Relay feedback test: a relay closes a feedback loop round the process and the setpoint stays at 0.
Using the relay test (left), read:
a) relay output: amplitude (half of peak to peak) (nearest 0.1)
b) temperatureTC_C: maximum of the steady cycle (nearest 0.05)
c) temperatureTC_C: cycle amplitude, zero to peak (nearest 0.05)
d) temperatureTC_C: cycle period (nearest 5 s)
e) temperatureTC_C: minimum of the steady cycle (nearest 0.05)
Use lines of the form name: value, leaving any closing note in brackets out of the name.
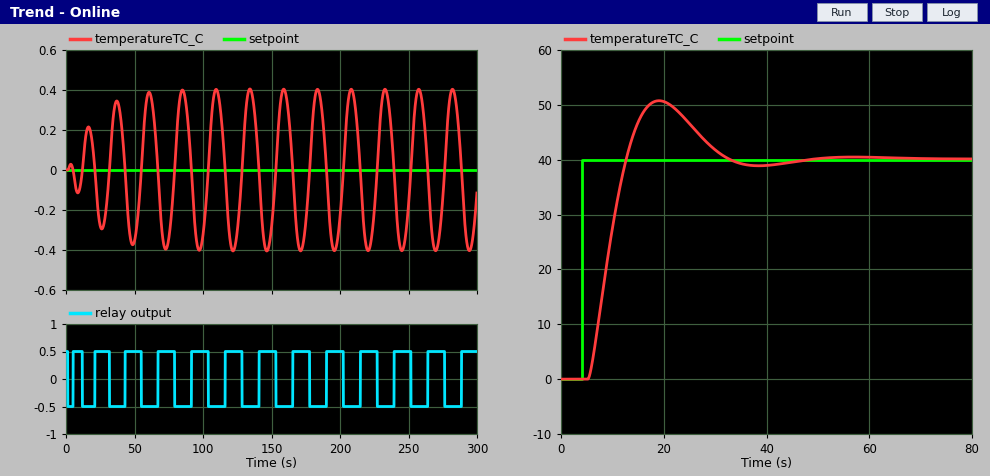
relay output: amplitude (half of peak to peak): 0.5
temperatureTC_C: maximum of the steady cycle: 0.40
temperatureTC_C: cycle amplitude, zero to peak: 0.40
temperatureTC_C: cycle period: 25 s
temperatureTC_C: minimum of the steady cycle: -0.40
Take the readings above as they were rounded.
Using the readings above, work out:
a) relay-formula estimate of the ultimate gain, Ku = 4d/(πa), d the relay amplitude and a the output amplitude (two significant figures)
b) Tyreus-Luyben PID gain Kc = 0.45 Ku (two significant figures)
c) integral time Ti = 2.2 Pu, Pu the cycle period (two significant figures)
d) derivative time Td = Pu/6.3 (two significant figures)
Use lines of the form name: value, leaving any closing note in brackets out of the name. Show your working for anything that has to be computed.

relay-formula estimate of the ultimate gain, Ku = 4d/(πa), d the relay amplitude and a the output amplitude: 4 × 0.5 / (π × 0.4) = 1.6
Tyreus-Luyben PID gain Kc = 0.45 Ku: 0.45 × 1.6 = 0.72
integral time Ti = 2.2 Pu, Pu the cycle period: 2.2 × 25 = 55 s
derivative time Td = Pu/6.3: 25 / 6.3 = 4.0 s
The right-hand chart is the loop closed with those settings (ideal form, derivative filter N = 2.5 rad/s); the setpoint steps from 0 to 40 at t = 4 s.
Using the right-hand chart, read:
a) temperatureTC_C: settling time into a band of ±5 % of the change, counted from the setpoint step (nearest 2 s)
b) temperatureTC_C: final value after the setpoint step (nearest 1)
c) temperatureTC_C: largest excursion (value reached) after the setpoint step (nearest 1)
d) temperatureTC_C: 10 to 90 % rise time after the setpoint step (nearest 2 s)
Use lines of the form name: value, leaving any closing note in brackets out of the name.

temperatureTC_C: settling time into a band of ±5 % of the change, counted from the setpoint step: 26 s
temperatureTC_C: final value after the setpoint step: 40
temperatureTC_C: largest excursion (value reached) after the setpoint step: 51
temperatureTC_C: 10 to 90 % rise time after the setpoint step: 6 s
